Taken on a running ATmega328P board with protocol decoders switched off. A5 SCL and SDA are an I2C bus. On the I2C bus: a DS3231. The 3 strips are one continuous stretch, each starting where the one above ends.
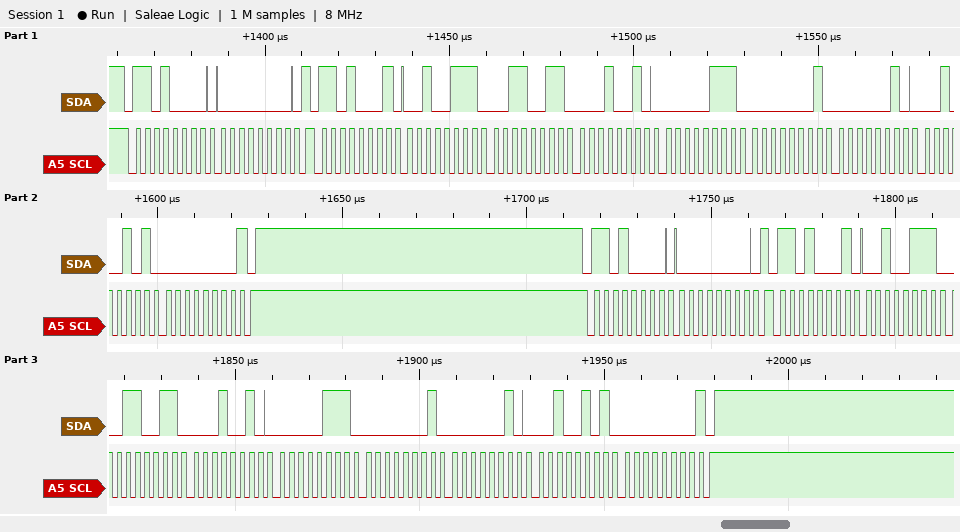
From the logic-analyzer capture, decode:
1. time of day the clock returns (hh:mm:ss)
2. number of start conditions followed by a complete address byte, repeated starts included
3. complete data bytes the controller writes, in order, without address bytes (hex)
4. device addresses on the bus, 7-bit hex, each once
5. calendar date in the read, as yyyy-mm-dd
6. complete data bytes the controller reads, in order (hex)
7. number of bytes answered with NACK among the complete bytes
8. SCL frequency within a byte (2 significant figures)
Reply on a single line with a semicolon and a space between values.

12:33:27; 4; 00 00; 0x68; 2025-02-01; 27 33 12 07 01 02 25 00 27 33 12 07 01 02 25 00; 2; 400 kHz
